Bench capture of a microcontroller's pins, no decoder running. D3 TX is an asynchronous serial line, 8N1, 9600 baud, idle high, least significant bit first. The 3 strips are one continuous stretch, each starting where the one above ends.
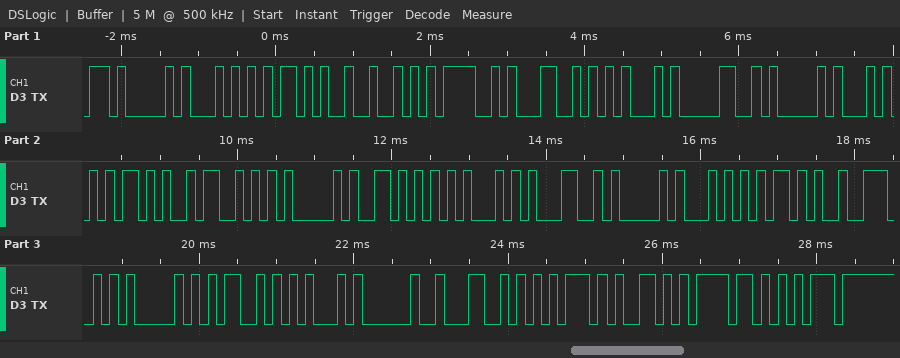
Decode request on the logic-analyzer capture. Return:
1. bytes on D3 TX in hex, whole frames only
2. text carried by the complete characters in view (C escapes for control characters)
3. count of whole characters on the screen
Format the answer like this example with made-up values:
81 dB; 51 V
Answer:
41 54 2B 52 4F 4C 45 30 41 54 2B 53 41 56 45 31 41 54 2B 4E 41 4D 45 20 4C 75 59 6F 75; "AT+ROLE0AT+SAVE1AT+NAME LuYou"; 29
